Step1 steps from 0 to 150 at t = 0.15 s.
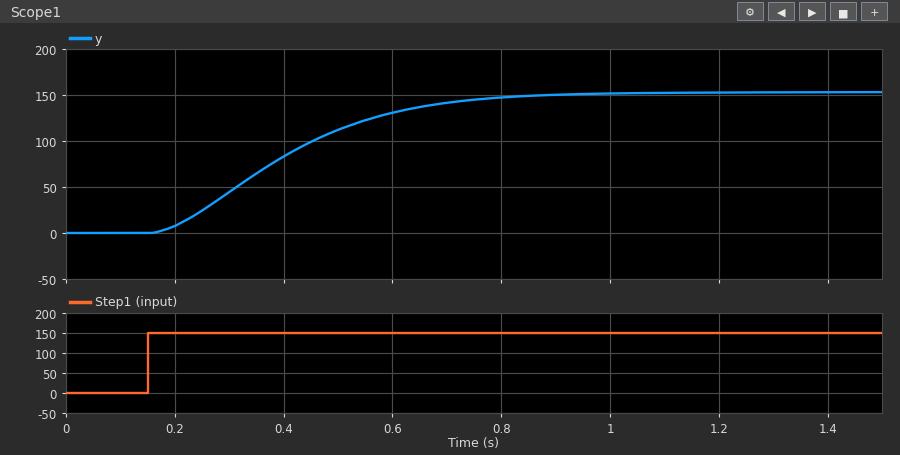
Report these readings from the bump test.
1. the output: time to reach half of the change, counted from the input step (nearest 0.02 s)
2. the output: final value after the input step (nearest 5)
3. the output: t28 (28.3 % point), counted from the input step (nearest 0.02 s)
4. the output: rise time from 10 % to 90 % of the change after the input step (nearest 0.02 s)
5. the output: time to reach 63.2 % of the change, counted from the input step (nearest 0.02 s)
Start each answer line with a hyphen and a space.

- 0.24 s
- 155
- 0.14 s
- 0.44 s
- 0.30 s
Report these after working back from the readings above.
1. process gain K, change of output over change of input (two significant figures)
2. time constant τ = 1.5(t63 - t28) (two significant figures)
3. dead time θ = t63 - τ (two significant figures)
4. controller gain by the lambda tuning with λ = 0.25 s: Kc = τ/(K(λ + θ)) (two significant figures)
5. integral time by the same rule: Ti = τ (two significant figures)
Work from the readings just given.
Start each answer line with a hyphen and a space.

- 1.0
- 0.24 s
- 0.060 s
- 0.77
- 0.24 s
